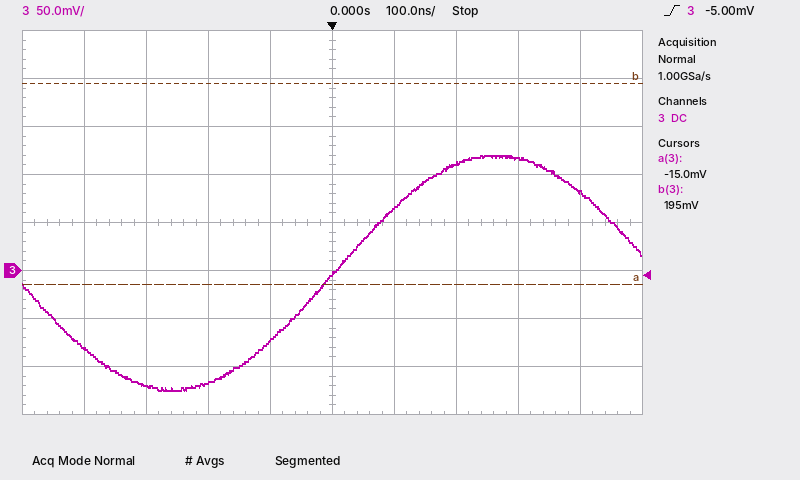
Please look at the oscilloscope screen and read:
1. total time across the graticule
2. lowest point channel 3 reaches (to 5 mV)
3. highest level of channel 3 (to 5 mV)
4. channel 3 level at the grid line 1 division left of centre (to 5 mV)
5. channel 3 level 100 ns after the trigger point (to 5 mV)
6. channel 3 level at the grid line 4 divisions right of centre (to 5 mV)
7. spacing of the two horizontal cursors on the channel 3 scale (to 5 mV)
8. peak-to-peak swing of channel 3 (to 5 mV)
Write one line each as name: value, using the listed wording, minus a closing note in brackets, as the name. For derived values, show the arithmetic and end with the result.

total time across the graticule: 1 µs
lowest point channel 3 reaches: -125 mV
highest level of channel 3: 120 mV
channel 3 level at the grid line 1 division left of centre: -75 mV
channel 3 level 100 ns after the trigger point: 65 mV
channel 3 level at the grid line 4 divisions right of centre: 80 mV
spacing of the two horizontal cursors on the channel 3 scale: 210 mV
peak-to-peak swing of channel 3: 120 mV − (-125 mV) = 245 mV
